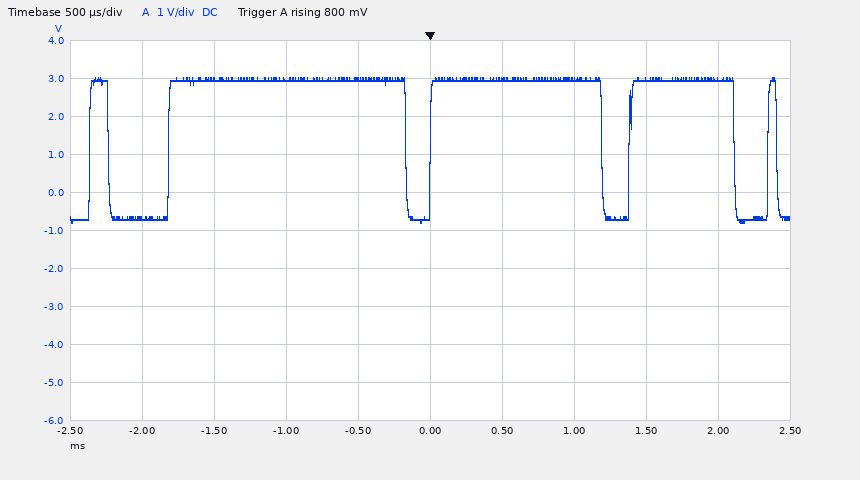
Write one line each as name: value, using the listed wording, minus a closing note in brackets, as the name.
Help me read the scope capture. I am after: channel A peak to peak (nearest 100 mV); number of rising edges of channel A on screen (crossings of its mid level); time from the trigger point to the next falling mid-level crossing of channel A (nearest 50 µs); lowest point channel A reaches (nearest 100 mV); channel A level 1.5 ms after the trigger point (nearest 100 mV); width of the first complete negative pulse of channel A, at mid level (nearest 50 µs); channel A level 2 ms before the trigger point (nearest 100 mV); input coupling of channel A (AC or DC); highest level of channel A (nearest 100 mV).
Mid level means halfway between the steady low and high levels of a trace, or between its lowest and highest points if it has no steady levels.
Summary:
channel A peak to peak: 3.8 V
number of rising edges of channel A on screen: 5
time from the trigger point to the next falling mid-level crossing of channel A: 1.20 ms
lowest point channel A reaches: -800 mV
channel A level 1.5 ms after the trigger point: 3.0 V
width of the first complete negative pulse of channel A, at mid level: 400 µs
channel A level 2 ms before the trigger point: -700 mV
input coupling of channel A: DC
highest level of channel A: 3.0 V
